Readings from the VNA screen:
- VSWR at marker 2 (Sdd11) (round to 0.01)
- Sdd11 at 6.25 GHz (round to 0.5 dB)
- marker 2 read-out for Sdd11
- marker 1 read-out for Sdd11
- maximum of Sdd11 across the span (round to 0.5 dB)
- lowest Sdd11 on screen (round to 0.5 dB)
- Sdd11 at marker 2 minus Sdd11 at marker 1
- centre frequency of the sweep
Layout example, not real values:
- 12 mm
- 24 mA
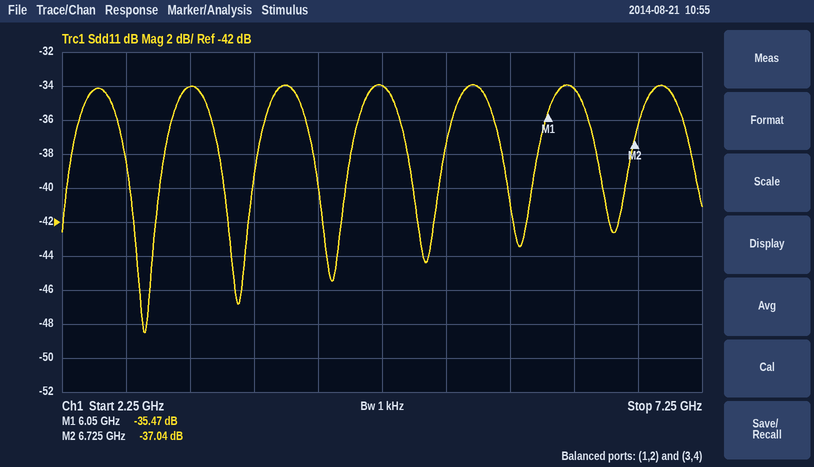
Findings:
- 1.03
- -34.0 dB
- -37.04 dB
- -35.47 dB
- -34.0 dB
- -48.5 dB
- -1.57 dB
- 4.75 GHz
